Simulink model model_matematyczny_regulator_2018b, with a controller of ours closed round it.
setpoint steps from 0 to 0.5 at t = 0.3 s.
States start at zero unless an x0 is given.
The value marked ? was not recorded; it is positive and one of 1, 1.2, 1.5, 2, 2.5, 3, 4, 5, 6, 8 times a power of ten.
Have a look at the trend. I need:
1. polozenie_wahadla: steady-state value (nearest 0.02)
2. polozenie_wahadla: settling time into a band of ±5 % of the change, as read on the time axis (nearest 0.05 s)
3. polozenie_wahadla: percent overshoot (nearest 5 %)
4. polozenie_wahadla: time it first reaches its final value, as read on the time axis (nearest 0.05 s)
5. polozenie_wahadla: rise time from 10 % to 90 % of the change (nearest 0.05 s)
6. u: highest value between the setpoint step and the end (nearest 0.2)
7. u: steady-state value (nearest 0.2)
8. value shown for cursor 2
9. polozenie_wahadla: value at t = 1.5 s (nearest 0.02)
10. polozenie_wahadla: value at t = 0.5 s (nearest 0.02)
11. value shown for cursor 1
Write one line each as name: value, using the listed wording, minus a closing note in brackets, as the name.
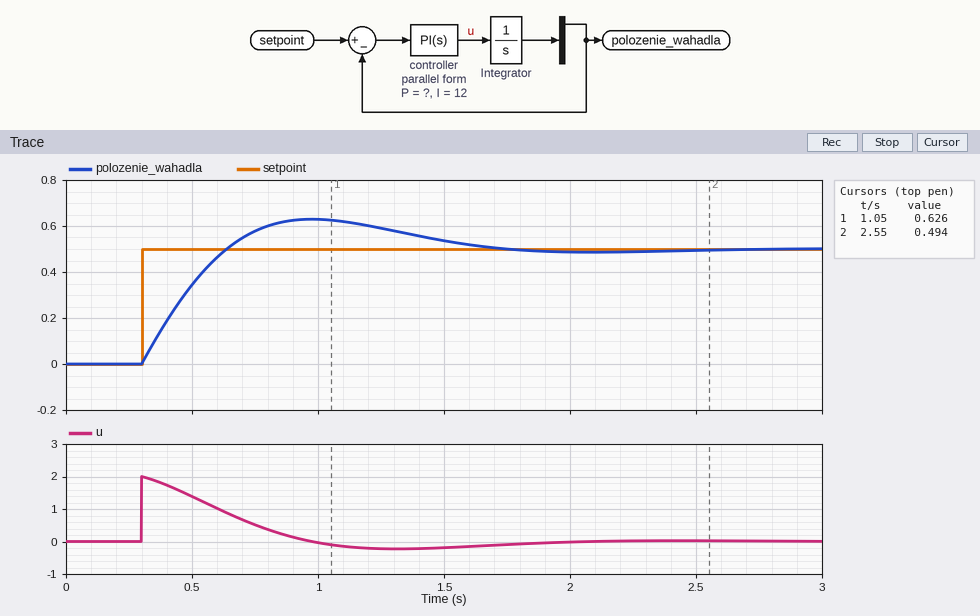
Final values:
polozenie_wahadla: steady-state value: 0.50
polozenie_wahadla: settling time into a band of ±5 % of the change, as read on the time axis: 1.55 s
polozenie_wahadla: percent overshoot: 25 %
polozenie_wahadla: time it first reaches its final value, as read on the time axis: 0.65 s
polozenie_wahadla: rise time from 10 % to 90 % of the change: 0.25 s
u: highest value between the setpoint step and the end: 2.0
u: steady-state value: 0.0
value shown for cursor 2: 0.494
polozenie_wahadla: value at t = 1.5 s: 0.54
polozenie_wahadla: value at t = 0.5 s: 0.34
value shown for cursor 1: 0.626
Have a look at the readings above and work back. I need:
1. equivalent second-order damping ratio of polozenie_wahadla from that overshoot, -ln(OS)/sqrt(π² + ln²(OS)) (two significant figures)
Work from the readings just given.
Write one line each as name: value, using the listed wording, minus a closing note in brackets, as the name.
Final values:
equivalent second-order damping ratio of polozenie_wahadla from that overshoot, -ln(OS)/sqrt(π² + ln²(OS)): 0.40
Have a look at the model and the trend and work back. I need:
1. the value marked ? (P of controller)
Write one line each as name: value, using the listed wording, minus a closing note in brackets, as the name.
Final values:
the value marked ?: 4
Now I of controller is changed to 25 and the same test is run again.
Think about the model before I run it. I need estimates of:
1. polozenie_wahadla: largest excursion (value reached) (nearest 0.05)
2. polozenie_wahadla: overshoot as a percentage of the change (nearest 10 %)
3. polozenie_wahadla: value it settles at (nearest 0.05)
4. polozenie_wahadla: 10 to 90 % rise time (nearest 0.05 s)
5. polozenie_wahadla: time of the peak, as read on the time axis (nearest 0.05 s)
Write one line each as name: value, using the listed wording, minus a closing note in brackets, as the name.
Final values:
polozenie_wahadla: largest excursion (value reached): 0.70
polozenie_wahadla: overshoot as a percentage of the change: 40 %
polozenie_wahadla: value it settles at: 0.50
polozenie_wahadla: 10 to 90 % rise time: 0.20 s
polozenie_wahadla: time of the peak, as read on the time axis: 0.80 s
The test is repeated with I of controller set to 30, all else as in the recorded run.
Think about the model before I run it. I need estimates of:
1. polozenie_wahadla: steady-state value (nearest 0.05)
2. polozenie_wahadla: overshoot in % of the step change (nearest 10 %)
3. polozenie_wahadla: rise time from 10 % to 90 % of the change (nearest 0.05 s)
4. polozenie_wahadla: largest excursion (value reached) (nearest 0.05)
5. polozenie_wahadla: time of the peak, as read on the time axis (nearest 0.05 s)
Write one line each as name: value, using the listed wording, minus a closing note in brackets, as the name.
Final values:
polozenie_wahadla: steady-state value: 0.50
polozenie_wahadla: overshoot in % of the step change: 40 %
polozenie_wahadla: rise time from 10 % to 90 % of the change: 0.20 s
polozenie_wahadla: largest excursion (value reached): 0.70
polozenie_wahadla: time of the peak, as read on the time axis: 0.75 s
